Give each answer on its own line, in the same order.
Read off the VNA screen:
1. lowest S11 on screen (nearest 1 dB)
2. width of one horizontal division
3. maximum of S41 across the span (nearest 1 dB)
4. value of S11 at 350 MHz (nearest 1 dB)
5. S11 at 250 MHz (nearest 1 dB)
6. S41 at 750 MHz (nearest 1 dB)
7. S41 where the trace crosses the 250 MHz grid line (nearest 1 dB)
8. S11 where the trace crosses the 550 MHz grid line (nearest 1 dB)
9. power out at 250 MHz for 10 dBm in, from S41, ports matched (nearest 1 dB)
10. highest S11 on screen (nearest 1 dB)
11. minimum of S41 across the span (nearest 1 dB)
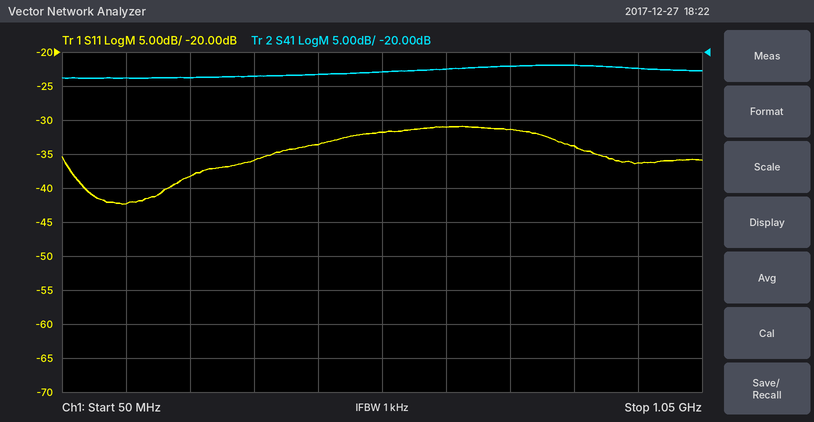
-42 dB
100 MHz
-22 dB
-36 dB
-38 dB
-22 dB
-24 dB
-32 dB
-14 dBm
-31 dB
-24 dB
